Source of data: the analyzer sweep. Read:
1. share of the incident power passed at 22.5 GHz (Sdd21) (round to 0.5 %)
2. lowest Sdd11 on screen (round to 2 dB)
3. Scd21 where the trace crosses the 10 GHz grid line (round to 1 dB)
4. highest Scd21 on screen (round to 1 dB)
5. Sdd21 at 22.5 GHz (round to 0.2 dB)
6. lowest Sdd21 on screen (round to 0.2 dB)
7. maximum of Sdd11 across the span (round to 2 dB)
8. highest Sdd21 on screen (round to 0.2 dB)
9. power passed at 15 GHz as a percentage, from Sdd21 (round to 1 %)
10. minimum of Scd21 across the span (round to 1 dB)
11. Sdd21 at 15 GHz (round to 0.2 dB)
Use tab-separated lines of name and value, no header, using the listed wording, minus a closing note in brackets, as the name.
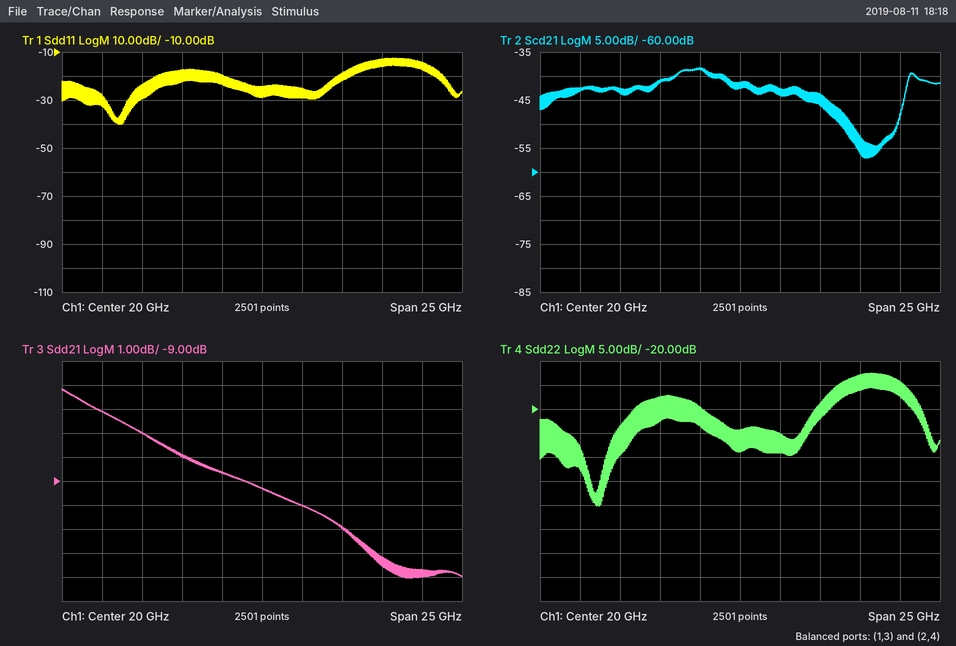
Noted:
share of the incident power passed at 22.5 GHz (Sdd21)	10.0 %
lowest Sdd11 on screen	-40 dB
Scd21 where the trace crosses the 10 GHz grid line	-43 dB
highest Scd21 on screen	-38 dB
Sdd21 at 22.5 GHz	-10.0 dB
lowest Sdd21 on screen	-13.0 dB
maximum of Sdd11 across the span	-12 dB
highest Sdd21 on screen	-5.2 dB
power passed at 15 GHz as a percentage, from Sdd21	16 %
minimum of Scd21 across the span	-57 dB
Sdd21 at 15 GHz	-8.0 dB
